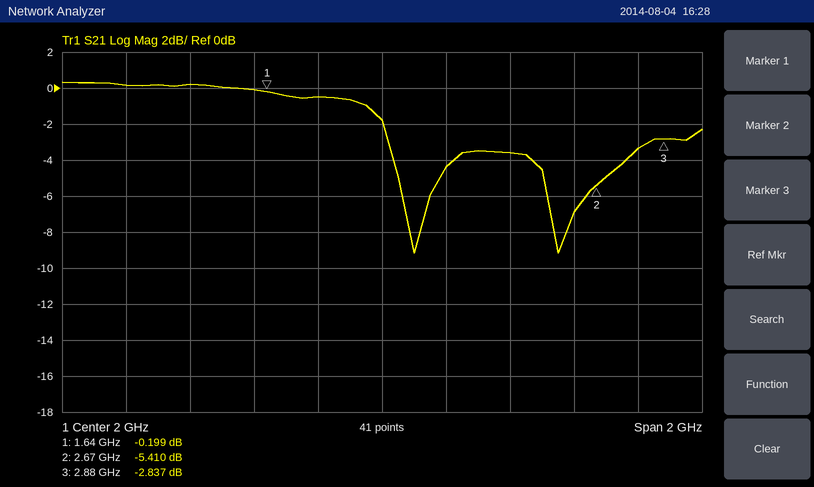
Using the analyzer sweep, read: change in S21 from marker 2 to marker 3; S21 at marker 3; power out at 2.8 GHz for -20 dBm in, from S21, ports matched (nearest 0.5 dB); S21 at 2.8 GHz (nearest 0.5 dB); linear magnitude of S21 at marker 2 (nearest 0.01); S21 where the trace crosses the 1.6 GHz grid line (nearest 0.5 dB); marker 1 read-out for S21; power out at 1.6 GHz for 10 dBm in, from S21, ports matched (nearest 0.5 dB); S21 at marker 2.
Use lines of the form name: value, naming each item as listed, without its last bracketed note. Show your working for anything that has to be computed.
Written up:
change in S21 from marker 2 to marker 3: -2.837 − (-5.41) = 2.573 dB
S21 at marker 3: -2.837 dB
power out at 2.8 GHz for -20 dBm in, from S21, ports matched: -20 dBm + (-3.5 dB) = -23.5 dBm
S21 at 2.8 GHz: -3.5 dB
linear magnitude of S21 at marker 2: 10^(-5.41/20) ≈ 0.54
S21 where the trace crosses the 1.6 GHz grid line: 0.0 dB
marker 1 read-out for S21: -0.199 dB
power out at 1.6 GHz for 10 dBm in, from S21, ports matched: 10 dBm + (0.0 dB) = 10.0 dBm
S21 at marker 2: -5.410 dB
